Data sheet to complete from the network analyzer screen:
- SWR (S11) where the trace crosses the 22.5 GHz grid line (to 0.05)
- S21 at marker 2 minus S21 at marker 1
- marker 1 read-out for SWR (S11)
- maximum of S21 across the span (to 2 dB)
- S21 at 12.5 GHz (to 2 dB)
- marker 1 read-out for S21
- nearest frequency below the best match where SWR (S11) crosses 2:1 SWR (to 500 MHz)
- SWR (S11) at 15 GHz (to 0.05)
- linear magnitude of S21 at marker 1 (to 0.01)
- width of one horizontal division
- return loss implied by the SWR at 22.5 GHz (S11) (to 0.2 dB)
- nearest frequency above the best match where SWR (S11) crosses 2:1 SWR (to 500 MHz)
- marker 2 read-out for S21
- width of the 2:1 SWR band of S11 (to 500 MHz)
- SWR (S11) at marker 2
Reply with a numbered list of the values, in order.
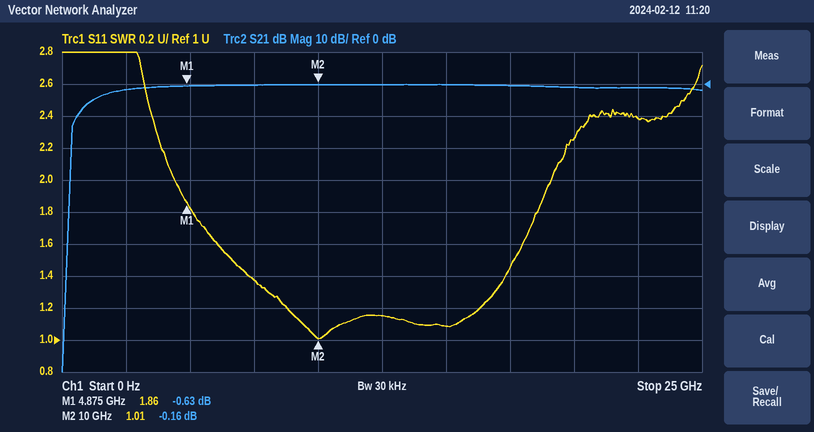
1. 2.40
2. 0.47 dB
3. 1.86
4. 0 dB
5. 0 dB
6. -0.63 dB
7. 4.5 GHz
8. 1.10
9. 0.93
10. 2.5 GHz
11. 7.8 dB
12. 19.0 GHz
13. -0.16 dB
14. 14.5 GHz
15. 1.01
